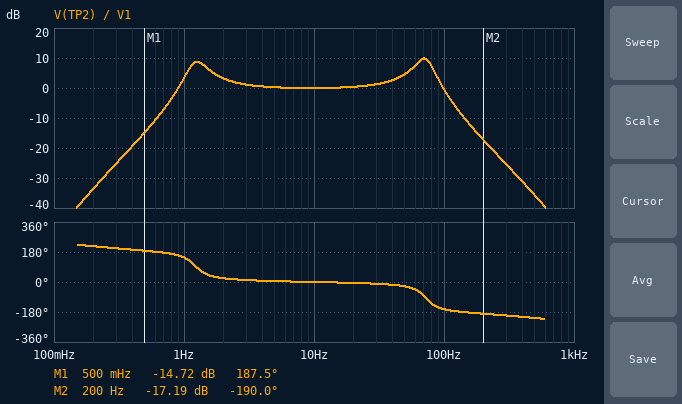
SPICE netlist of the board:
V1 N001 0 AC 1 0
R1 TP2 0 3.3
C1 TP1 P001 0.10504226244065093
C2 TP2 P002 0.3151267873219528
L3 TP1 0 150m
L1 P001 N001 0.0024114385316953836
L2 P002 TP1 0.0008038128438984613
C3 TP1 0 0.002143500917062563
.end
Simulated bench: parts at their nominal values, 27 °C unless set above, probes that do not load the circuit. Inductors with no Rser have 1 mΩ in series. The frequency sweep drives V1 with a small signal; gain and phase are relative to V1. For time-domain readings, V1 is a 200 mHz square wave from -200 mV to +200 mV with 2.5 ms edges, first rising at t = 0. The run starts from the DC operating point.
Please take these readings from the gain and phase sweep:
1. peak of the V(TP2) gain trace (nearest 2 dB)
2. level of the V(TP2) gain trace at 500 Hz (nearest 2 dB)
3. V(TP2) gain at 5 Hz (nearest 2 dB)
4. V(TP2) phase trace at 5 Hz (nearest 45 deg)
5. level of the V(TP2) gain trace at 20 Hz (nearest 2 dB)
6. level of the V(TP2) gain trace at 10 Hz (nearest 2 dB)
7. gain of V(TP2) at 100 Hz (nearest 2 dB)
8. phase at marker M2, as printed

10 dB
-36 dB
0 dB
0 deg
0 dB
0 dB
0 dB
-190.0 deg
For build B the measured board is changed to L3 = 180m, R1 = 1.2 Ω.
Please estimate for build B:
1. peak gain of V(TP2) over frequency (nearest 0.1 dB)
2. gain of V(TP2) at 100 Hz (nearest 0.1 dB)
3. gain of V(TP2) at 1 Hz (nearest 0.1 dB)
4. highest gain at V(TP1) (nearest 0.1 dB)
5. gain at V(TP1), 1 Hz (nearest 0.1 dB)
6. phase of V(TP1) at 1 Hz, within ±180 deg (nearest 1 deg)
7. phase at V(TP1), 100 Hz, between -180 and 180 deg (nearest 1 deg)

1.3 dB
-2.3 dB
-1.3 dB
1.6 dB
-0.6 dB
83 deg
-118 deg
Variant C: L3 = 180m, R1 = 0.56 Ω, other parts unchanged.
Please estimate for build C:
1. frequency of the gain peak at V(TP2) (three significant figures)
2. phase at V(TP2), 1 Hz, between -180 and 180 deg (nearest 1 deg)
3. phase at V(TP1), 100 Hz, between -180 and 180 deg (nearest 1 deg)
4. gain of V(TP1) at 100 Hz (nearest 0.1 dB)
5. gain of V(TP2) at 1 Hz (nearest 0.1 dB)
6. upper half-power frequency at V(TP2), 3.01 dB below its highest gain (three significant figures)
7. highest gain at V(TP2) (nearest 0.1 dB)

10.4 Hz
97 deg
-78 deg
-3.7 dB
-7.7 dB
38.8 Hz
0 dB
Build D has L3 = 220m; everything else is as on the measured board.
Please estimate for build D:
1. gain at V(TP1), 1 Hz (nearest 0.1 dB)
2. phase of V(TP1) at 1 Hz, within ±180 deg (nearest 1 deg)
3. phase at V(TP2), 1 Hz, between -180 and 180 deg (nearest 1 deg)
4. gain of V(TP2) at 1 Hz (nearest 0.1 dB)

7.0 dB
90 deg
98 deg
6.9 dB
